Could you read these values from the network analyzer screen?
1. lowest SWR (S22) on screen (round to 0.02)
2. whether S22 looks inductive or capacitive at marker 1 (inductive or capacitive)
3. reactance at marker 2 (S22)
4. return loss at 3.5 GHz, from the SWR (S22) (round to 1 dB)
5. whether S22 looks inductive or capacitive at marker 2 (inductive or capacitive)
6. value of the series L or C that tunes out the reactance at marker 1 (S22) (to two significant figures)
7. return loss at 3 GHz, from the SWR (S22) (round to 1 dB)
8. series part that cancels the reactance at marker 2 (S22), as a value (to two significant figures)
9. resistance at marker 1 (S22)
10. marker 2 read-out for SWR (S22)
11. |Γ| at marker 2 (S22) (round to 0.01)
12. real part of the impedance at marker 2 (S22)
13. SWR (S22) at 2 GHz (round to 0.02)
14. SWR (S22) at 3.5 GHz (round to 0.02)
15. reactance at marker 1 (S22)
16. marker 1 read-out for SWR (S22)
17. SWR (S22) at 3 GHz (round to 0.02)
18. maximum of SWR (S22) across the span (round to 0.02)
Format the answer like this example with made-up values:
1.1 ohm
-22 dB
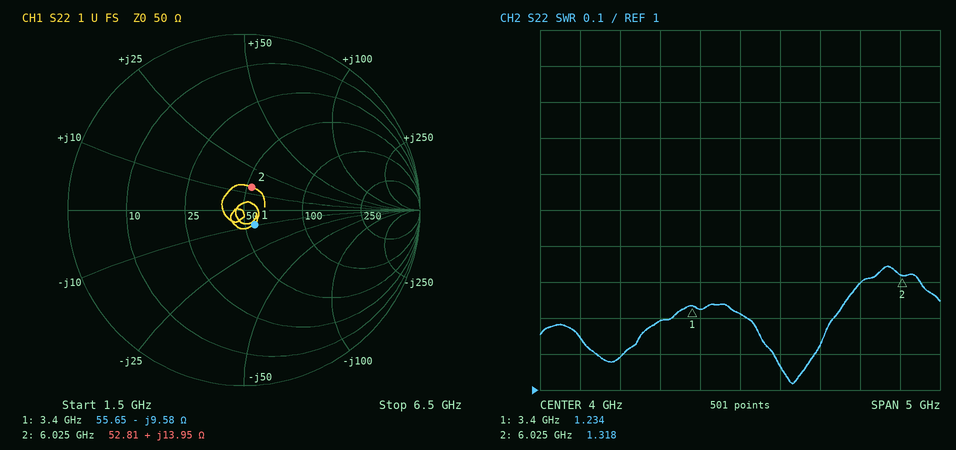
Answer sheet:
1.02
capacitive
+13.95 Ω
20 dB
inductive
450 pH
21 dB
1.9 pF
55.65 Ω
1.318
0.14
52.81 Ω
1.14
1.22
-9.58 Ω
1.234
1.20
1.34
